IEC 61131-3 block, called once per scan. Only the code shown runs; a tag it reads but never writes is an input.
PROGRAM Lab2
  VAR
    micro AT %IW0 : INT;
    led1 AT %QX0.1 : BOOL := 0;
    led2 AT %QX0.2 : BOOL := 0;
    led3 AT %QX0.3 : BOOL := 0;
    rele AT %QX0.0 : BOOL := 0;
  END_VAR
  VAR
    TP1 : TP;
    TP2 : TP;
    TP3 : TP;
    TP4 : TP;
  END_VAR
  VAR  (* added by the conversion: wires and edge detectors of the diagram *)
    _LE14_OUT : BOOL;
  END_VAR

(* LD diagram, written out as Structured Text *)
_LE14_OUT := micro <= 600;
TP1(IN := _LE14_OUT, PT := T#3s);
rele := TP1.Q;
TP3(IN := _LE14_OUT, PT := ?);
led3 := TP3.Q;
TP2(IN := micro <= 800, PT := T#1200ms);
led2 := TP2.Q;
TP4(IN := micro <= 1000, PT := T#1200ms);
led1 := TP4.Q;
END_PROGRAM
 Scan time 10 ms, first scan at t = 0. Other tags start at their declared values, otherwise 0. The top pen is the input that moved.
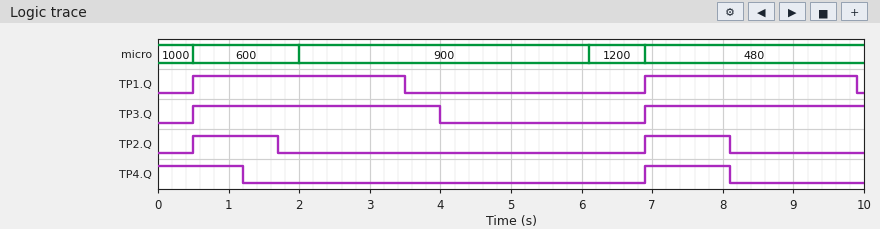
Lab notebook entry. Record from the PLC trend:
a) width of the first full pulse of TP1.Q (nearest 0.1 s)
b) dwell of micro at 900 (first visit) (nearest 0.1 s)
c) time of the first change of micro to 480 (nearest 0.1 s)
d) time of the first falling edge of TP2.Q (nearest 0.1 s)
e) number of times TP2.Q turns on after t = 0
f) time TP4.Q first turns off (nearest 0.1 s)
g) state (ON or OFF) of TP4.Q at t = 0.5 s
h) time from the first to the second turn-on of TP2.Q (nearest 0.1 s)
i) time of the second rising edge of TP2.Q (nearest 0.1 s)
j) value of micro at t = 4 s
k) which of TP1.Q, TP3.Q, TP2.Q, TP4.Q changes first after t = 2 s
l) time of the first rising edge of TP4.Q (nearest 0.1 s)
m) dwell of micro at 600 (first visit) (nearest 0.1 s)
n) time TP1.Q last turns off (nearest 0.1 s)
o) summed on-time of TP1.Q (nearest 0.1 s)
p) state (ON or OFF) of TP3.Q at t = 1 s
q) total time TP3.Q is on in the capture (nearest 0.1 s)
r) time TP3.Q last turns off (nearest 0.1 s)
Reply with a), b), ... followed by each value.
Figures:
a) 3.0 s
b) 4.1 s
c) 6.9 s
d) 1.7 s
e) 2
f) 1.2 s
g) ON
h) 6.4 s
i) 6.9 s
j) 900
k) TP1.Q
l) 6.9 s
m) 1.5 s
n) 9.9 s
o) 6.0 s
p) ON
q) 6.6 s
r) 4.0 s
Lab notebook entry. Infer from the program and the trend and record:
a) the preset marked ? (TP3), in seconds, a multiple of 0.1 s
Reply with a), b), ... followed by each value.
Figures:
a) 3.5 s
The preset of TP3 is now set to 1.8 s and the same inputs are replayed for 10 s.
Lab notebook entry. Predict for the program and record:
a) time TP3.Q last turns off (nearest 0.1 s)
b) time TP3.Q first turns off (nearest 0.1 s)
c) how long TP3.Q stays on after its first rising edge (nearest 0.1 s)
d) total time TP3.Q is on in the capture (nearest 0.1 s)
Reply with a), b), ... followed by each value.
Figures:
a) 8.7 s
b) 2.3 s
c) 1.8 s
d) 3.6 s
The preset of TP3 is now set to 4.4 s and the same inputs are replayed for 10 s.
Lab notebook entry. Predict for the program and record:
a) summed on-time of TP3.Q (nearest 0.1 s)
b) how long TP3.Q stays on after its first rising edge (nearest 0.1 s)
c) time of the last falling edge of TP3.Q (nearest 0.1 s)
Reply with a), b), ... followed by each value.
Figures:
a) 7.5 s
b) 4.4 s
c) 4.9 s
